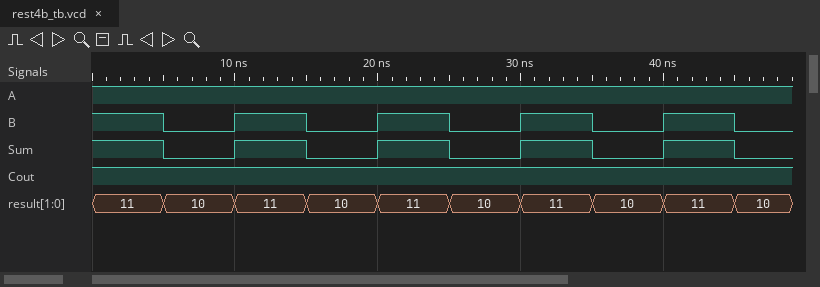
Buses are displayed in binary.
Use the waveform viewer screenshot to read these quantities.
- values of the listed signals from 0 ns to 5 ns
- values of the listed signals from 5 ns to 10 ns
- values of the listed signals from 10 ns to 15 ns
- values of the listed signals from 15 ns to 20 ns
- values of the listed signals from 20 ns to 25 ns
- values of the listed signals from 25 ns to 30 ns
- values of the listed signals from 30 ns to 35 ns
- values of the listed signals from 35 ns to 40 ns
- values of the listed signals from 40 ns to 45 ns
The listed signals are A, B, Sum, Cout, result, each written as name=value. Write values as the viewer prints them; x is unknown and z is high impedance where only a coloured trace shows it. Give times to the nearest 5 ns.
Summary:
A=1, B=1, Sum=1, Cout=1, result=11
A=1, B=0, Sum=0, Cout=1, result=10
A=1, B=1, Sum=1, Cout=1, result=11
A=1, B=0, Sum=0, Cout=1, result=10
A=1, B=1, Sum=1, Cout=1, result=11
A=1, B=0, Sum=0, Cout=1, result=10
A=1, B=1, Sum=1, Cout=1, result=11
A=1, B=0, Sum=0, Cout=1, result=10
A=1, B=1, Sum=1, Cout=1, result=11
